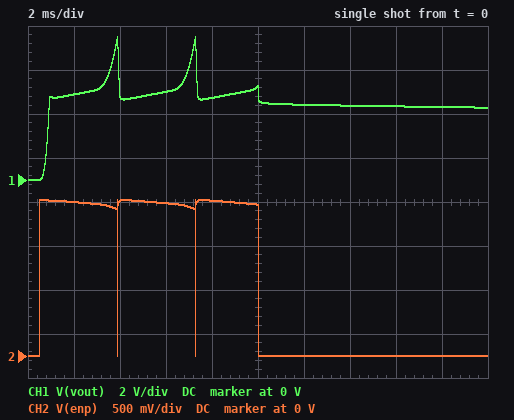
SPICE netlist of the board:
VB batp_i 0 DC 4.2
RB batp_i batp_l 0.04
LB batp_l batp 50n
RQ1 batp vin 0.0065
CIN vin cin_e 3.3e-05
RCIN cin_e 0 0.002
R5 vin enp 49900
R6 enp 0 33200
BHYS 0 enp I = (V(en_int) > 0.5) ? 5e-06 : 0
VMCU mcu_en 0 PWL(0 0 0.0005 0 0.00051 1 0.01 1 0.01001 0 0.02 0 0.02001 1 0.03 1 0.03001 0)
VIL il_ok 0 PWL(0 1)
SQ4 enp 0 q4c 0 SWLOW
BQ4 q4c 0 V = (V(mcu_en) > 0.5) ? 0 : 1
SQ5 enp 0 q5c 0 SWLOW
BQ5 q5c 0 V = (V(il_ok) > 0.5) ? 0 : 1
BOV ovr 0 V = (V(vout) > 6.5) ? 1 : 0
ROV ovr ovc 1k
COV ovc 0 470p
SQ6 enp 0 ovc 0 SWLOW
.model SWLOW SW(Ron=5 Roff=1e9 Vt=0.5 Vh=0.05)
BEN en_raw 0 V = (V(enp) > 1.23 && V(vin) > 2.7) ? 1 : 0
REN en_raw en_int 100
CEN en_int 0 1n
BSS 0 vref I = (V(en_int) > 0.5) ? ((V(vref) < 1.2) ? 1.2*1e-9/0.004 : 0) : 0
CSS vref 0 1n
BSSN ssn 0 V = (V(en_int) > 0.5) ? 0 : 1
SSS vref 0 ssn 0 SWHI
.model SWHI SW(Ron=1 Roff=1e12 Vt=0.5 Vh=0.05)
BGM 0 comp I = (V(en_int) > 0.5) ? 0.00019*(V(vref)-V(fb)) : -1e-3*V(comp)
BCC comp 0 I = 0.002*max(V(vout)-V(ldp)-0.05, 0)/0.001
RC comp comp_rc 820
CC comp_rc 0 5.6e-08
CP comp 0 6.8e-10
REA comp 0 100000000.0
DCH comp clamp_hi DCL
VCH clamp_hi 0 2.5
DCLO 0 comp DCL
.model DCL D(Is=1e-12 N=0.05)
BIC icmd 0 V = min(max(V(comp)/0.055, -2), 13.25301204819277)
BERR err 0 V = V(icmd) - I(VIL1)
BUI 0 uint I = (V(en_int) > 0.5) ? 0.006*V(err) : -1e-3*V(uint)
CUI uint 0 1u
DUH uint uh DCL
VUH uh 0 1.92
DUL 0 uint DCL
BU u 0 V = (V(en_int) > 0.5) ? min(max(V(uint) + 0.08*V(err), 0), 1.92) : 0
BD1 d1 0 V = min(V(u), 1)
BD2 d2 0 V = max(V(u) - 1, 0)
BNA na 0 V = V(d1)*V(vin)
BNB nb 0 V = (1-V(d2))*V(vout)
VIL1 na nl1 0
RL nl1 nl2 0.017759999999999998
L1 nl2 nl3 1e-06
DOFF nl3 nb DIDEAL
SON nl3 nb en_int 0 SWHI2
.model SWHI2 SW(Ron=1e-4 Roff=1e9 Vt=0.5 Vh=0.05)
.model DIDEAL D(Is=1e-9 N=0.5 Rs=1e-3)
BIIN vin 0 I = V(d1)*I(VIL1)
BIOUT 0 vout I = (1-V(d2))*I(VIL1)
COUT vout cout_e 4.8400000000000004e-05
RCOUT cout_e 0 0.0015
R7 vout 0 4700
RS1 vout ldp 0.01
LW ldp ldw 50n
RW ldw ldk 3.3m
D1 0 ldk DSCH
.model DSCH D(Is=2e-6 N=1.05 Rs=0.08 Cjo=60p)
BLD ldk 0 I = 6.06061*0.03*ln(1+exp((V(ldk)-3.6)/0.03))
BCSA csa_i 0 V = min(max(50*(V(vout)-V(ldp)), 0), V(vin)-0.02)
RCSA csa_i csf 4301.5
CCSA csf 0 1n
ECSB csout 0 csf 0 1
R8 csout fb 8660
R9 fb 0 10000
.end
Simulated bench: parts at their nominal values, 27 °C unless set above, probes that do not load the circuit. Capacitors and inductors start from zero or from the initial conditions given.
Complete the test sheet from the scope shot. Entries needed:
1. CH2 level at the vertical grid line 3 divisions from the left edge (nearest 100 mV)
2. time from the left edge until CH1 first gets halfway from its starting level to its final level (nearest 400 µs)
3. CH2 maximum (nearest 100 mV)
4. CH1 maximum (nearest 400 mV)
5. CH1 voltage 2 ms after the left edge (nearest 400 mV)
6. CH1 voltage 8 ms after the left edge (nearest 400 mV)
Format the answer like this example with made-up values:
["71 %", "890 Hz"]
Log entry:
["1.7 V", "800 µs", "1.8 V", "6.4 V", "4.0 V", "3.6 V"]
